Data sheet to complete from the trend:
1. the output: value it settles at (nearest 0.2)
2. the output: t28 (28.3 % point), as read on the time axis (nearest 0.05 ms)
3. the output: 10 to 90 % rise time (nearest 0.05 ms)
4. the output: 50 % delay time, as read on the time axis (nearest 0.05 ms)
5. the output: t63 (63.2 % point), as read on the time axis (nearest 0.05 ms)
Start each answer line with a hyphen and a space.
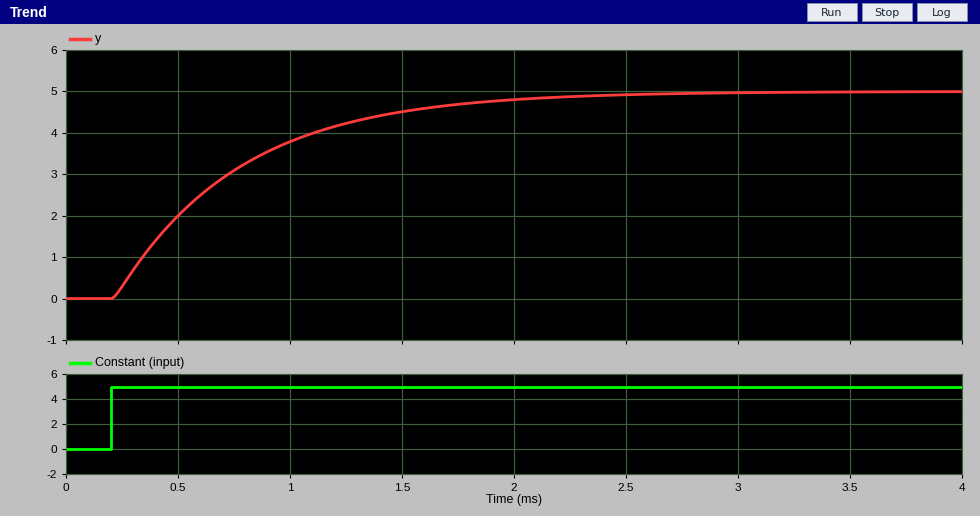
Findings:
- 5.0
- 0.40 ms
- 1.20 ms
- 0.60 ms
- 0.75 ms
